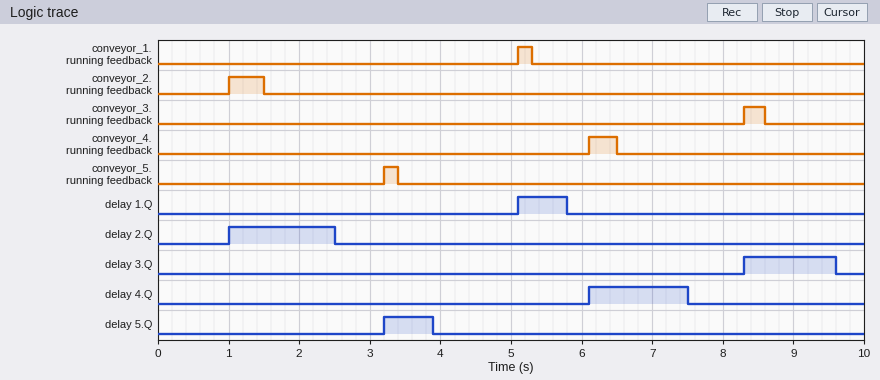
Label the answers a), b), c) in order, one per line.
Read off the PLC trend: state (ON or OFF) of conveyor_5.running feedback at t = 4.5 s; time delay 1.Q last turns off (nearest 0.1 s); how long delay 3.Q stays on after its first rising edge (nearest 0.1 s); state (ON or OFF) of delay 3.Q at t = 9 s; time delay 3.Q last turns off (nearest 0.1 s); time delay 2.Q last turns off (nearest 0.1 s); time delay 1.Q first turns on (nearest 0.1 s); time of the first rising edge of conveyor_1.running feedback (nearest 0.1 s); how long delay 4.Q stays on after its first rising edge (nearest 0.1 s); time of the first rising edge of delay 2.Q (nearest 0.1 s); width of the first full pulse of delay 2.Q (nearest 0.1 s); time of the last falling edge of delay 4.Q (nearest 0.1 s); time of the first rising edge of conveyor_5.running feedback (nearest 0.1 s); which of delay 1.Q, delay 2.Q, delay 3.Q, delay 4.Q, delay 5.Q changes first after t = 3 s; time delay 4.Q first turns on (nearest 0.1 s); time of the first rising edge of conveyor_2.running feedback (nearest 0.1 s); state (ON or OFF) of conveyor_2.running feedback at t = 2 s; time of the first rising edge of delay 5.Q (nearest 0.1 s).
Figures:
a) OFF
b) 5.8 s
c) 1.3 s
d) ON
e) 9.6 s
f) 2.5 s
g) 5.1 s
h) 5.1 s
i) 1.4 s
j) 1.0 s
k) 1.5 s
l) 7.5 s
m) 3.2 s
n) delay 5.Q
o) 6.1 s
p) 1.0 s
q) OFF
r) 3.2 s
